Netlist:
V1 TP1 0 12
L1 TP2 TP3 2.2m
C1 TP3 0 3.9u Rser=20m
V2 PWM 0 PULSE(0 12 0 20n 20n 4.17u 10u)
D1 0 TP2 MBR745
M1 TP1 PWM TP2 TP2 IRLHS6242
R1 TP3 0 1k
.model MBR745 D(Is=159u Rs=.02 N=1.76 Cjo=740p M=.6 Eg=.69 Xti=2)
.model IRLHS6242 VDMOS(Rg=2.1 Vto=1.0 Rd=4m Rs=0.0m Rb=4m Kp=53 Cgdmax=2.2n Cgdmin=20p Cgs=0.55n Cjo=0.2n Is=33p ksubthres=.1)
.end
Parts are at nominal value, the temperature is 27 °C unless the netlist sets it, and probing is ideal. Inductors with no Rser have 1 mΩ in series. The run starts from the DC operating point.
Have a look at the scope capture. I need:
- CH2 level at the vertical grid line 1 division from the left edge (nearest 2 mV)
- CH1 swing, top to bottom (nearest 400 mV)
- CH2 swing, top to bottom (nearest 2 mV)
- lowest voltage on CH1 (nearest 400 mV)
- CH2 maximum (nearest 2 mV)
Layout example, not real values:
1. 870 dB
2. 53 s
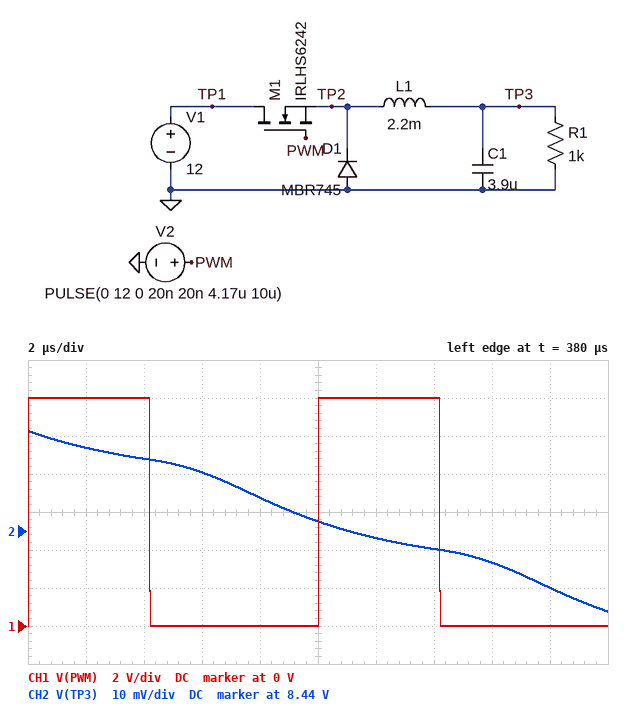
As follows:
1. 8.462 V
2. 12.0 V
3. 48 mV
4. 0 V
5. 8.466 V
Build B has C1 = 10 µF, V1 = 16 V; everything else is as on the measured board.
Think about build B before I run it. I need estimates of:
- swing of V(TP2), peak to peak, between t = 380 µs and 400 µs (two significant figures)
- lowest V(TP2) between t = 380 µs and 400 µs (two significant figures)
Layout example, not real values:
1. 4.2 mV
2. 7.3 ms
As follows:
1. 11 V
2. -320 mV
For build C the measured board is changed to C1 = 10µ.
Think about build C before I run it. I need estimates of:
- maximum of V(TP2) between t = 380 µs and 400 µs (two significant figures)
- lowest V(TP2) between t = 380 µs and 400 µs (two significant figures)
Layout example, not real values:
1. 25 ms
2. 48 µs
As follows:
1. 11 V
2. -320 mV
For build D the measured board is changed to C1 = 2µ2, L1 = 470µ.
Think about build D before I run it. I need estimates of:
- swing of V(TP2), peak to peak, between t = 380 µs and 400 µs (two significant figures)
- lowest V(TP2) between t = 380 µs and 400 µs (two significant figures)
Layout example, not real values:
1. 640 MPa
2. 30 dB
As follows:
1. 13 V
2. -230 mV
